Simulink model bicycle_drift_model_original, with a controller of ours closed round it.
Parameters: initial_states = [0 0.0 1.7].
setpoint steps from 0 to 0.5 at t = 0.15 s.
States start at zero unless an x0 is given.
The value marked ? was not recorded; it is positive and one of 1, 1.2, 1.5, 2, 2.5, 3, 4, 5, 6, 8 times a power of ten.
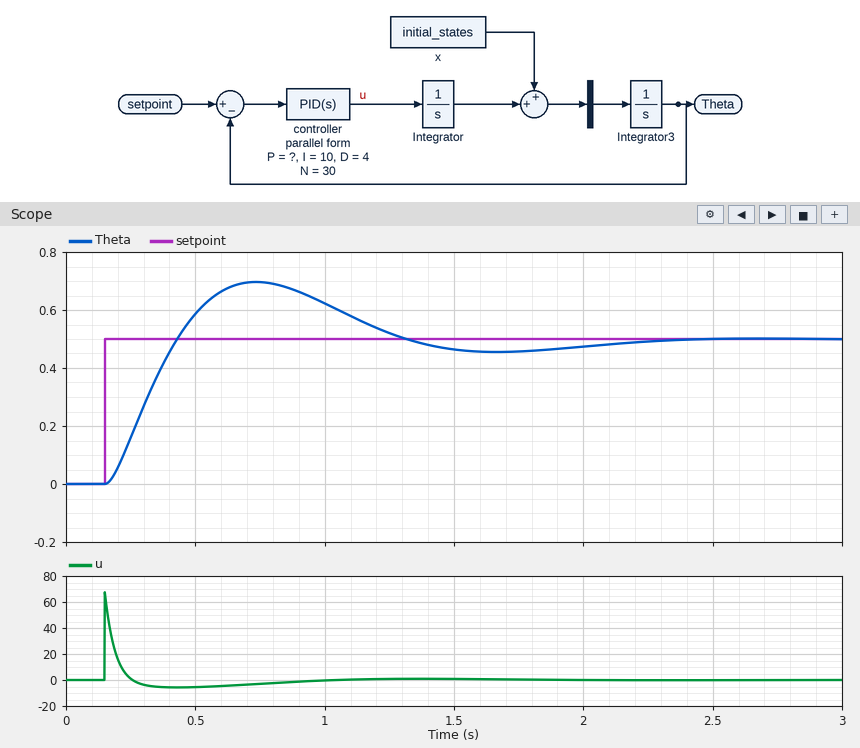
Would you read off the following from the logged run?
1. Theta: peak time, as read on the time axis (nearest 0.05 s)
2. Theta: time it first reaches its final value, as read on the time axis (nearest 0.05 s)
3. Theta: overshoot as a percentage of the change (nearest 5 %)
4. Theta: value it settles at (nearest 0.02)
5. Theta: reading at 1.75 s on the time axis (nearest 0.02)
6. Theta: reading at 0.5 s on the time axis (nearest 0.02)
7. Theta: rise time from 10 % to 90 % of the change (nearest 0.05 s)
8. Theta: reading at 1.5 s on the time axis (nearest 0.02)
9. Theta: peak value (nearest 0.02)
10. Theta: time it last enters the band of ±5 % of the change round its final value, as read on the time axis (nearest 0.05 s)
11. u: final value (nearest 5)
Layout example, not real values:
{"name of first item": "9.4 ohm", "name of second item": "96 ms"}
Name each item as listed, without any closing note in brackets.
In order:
{"Theta: peak time, as read on the time axis": "0.75 s", "Theta: time it first reaches its final value, as read on the time axis": "0.45 s", "Theta: overshoot as a percentage of the change": "40 %", "Theta: value it settles at": "0.50", "Theta: reading at 1.75 s on the time axis": "0.46", "Theta: reading at 0.5 s on the time axis": "0.58", "Theta: rise time from 10 % to 90 % of the change": "0.20 s", "Theta: reading at 1.5 s on the time axis": "0.46", "Theta: peak value": "0.70", "Theta: time it last enters the band of ±5 % of the change round its final value, as read on the time axis": "2.00 s", "u: final value": "0"}
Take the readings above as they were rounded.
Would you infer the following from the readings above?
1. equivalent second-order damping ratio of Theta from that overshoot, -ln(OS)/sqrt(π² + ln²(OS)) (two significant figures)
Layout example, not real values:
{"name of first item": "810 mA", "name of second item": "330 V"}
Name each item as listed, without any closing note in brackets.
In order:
{"equivalent second-order damping ratio of Theta from that overshoot, -ln(OS)/sqrt(π² + ln²(OS))": "0.28"}
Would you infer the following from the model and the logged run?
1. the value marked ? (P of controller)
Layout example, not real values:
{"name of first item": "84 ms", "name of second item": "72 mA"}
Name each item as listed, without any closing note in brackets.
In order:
{"the value marked ?": "15"}
